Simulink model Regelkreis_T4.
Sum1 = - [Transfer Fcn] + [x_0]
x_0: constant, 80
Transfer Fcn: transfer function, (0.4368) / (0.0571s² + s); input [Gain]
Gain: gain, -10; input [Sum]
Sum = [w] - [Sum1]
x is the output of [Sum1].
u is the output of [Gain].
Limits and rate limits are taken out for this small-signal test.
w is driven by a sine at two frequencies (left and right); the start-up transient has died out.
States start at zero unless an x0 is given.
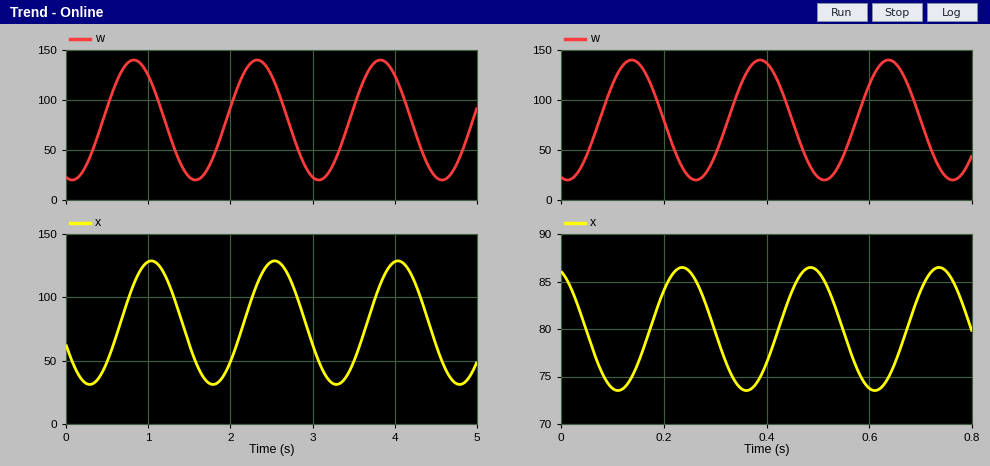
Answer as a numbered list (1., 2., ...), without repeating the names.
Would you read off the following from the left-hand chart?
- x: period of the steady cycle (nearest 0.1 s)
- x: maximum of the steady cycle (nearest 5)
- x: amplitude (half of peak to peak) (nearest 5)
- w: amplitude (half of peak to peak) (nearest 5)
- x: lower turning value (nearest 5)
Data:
1. 1.5 s
2. 130
3. 50
4. 60
5. 30
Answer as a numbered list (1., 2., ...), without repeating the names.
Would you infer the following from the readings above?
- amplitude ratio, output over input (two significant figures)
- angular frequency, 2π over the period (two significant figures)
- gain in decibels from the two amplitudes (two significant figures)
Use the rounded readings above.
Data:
1. 0.83
2. 4.2 rad/s
3. -1.6 dB
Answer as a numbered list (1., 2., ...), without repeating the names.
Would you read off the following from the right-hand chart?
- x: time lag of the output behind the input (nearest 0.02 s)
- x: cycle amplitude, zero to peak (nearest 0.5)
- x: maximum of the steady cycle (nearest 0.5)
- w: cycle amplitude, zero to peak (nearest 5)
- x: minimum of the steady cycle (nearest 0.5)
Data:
1. 0.10 s
2. 6.5
3. 86.5
4. 60
5. 73.5
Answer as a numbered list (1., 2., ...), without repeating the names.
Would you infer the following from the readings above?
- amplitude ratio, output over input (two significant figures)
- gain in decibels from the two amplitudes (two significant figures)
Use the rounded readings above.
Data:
1. 0.11
2. -19 dB
